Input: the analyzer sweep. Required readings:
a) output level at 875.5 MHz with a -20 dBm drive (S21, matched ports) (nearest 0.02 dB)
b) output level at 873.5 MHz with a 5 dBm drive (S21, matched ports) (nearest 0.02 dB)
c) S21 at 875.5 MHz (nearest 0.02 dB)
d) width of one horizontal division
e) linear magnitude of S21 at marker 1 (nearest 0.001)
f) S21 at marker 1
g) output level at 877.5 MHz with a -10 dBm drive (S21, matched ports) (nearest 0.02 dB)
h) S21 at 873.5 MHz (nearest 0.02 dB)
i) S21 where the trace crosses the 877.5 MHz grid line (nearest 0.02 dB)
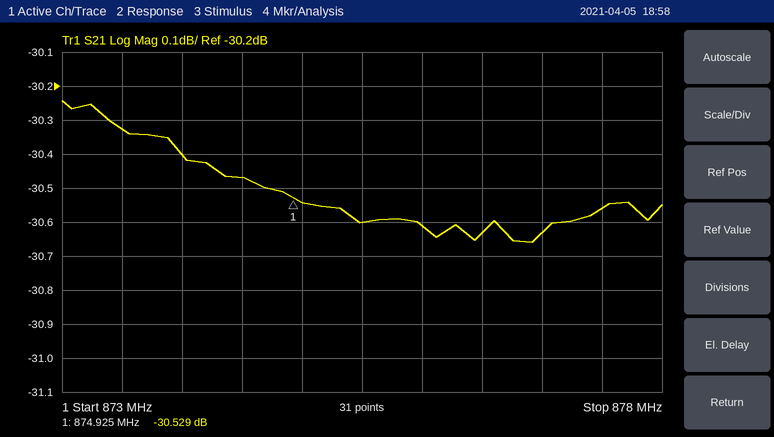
-50.60 dBm
-25.32 dBm
-30.60 dB
500 kHz
0.030
-30.529 dB
-40.56 dBm
-30.32 dB
-30.56 dB
